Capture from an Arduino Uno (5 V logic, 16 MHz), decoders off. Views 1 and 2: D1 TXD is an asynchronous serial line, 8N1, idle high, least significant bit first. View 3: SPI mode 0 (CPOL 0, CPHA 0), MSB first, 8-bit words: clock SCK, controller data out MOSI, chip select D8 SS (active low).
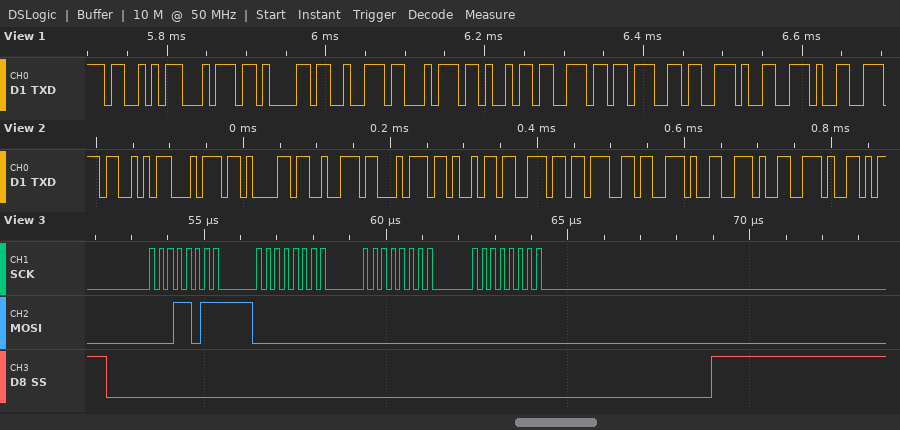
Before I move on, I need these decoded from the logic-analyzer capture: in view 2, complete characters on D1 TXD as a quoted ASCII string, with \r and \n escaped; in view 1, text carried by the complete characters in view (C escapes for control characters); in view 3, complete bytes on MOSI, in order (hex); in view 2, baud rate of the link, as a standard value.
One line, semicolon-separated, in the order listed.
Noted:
"Starting..."; "Starting.."; 1B 00 00 00; 115200 baud
